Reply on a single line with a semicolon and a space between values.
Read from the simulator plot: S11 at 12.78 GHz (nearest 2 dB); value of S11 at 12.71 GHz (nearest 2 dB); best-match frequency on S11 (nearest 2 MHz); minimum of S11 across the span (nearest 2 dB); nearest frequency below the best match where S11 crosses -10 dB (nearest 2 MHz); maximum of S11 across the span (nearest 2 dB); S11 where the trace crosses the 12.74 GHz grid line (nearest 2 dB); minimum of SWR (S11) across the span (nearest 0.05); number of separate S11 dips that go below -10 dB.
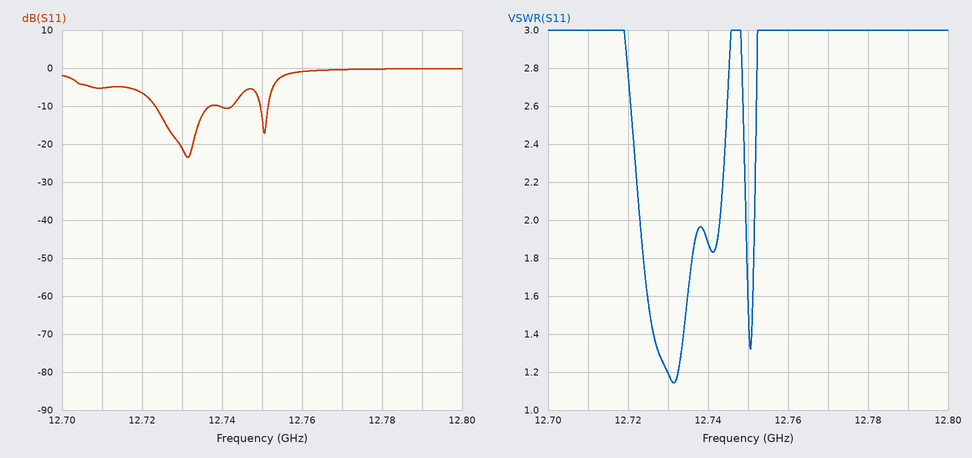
0 dB; -6 dB; 12.732 GHz; -24 dB; 12.724 GHz; 0 dB; -10 dB; 1.15; 2
